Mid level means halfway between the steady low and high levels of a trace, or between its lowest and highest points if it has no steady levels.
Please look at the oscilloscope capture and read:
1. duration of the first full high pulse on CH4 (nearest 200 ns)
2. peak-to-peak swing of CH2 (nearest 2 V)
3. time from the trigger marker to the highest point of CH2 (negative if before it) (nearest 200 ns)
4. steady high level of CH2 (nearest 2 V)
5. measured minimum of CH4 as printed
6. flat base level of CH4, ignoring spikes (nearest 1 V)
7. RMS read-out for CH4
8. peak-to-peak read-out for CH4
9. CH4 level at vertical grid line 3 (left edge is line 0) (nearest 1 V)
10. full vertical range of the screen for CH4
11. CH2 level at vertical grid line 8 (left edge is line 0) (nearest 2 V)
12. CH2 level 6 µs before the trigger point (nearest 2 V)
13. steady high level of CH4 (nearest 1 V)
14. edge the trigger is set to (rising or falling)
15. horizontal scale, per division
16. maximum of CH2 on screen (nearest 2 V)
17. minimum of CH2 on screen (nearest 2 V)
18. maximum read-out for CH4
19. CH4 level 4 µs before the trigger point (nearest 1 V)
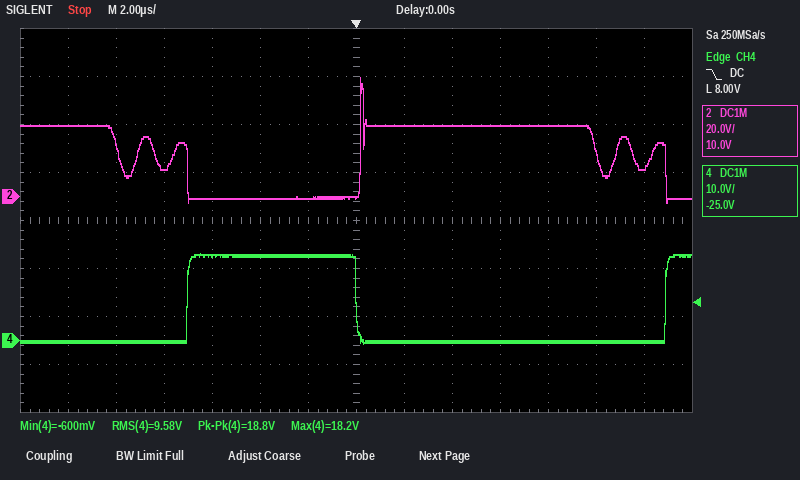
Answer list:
7.0 µs
52 V
+200 ns
30 V
-600 mV
0 V
9.58 V
18.8 V
0 V
80 V
30 V
0 V
18 V
falling
2 µs
50 V
-2 V
18.2 V
18 V
